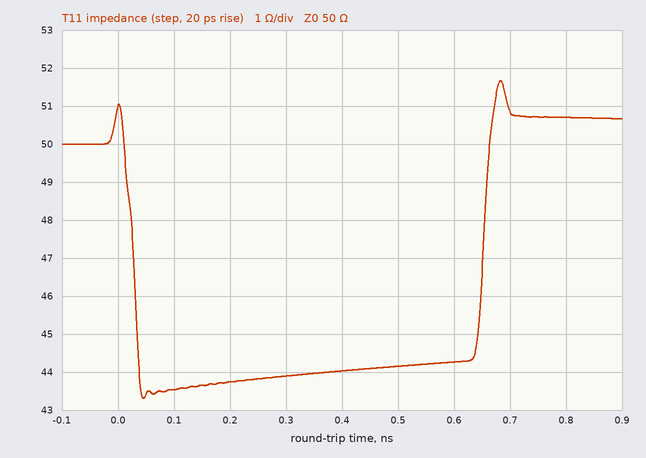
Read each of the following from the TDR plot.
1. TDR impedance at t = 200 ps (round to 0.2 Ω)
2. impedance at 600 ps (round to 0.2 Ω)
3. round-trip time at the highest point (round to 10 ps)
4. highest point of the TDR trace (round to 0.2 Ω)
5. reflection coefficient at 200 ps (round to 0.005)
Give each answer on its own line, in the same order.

43.8 Ω
44.2 Ω
680 ps
51.6 Ω
-0.065
